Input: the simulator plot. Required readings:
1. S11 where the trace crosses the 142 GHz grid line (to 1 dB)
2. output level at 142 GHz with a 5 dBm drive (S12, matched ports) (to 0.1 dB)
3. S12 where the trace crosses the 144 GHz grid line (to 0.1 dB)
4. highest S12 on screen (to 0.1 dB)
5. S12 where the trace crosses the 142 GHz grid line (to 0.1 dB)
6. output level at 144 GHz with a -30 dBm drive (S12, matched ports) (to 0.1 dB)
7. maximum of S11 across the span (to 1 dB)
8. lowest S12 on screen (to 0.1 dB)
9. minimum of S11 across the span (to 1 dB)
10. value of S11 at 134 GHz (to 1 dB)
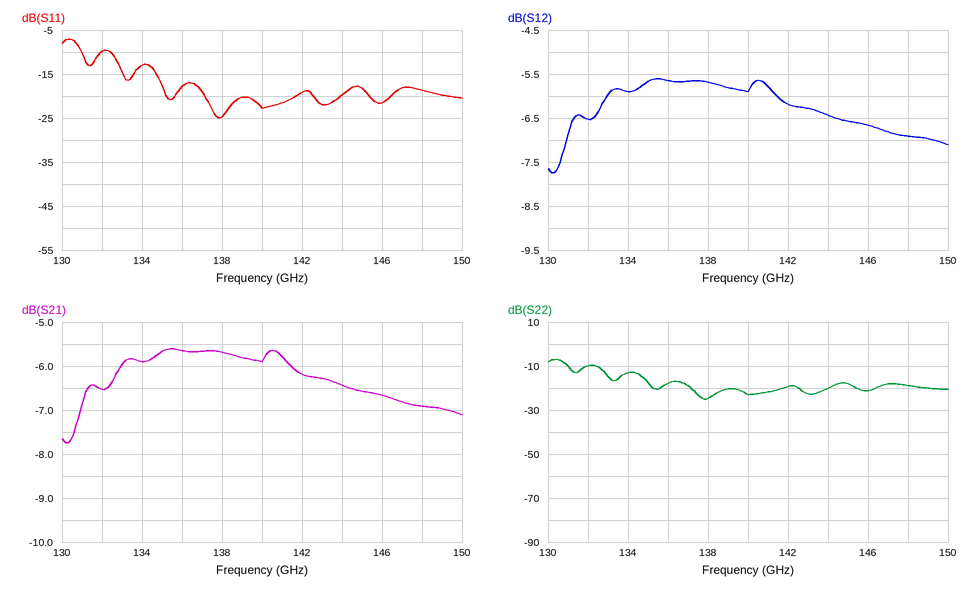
-19 dB
-1.2 dBm
-6.4 dB
-5.6 dB
-6.2 dB
-36.4 dBm
-7 dB
-7.7 dB
-25 dB
-13 dB
